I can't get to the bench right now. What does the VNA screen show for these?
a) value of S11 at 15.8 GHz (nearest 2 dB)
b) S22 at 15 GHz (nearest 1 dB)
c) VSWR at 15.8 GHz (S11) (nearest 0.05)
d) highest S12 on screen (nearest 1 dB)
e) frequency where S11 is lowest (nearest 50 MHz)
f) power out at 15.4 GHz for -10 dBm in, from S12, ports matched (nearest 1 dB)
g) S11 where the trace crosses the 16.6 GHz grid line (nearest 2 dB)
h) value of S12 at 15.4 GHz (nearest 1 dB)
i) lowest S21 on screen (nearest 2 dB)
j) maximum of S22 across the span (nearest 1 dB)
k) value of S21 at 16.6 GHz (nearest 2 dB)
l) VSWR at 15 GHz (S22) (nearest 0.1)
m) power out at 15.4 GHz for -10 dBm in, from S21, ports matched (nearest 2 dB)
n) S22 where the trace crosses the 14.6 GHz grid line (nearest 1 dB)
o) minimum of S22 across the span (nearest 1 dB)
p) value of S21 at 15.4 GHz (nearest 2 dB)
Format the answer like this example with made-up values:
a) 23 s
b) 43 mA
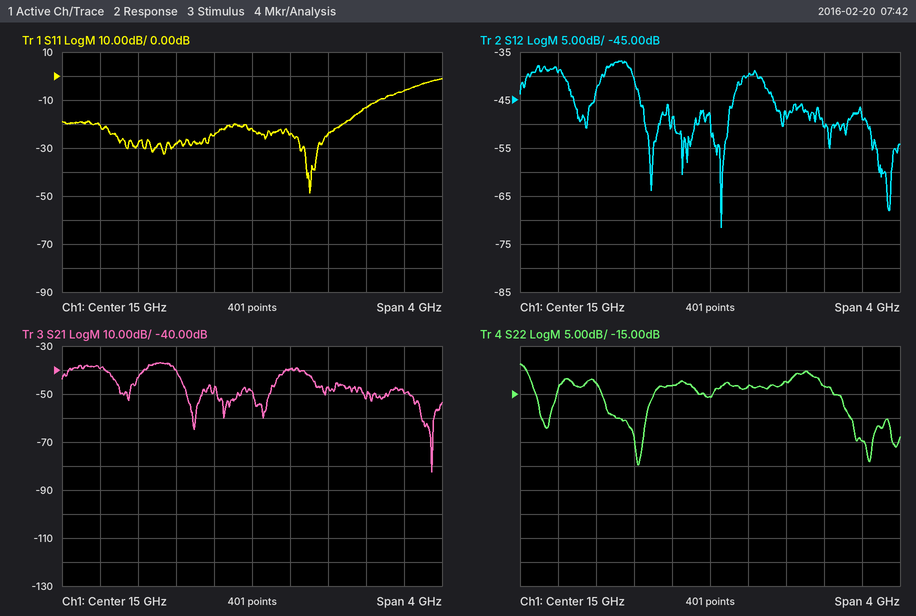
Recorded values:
a) -24 dB
b) -16 dB
c) 1.15
d) -37 dB
e) 15.60 GHz
f) -50 dBm
g) -6 dB
h) -40 dB
i) -82 dB
j) -9 dB
k) -50 dB
l) 1.4
m) -50 dBm
n) -13 dB
o) -30 dB
p) -40 dB
